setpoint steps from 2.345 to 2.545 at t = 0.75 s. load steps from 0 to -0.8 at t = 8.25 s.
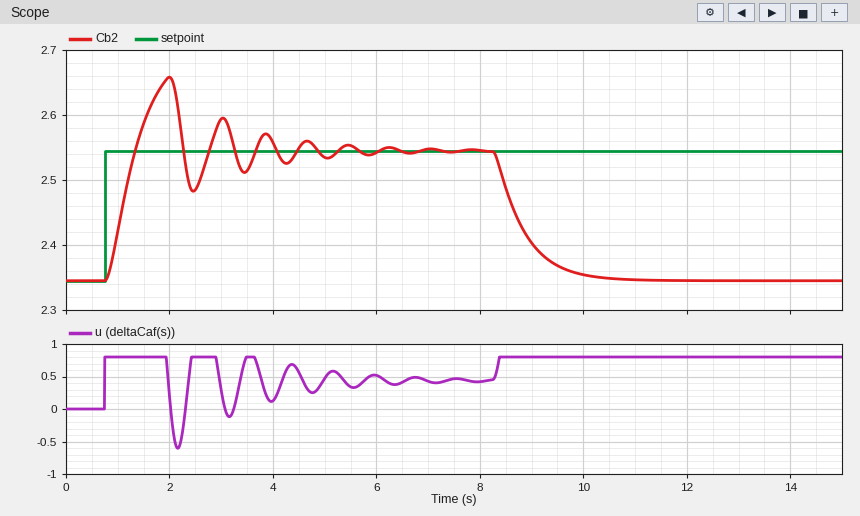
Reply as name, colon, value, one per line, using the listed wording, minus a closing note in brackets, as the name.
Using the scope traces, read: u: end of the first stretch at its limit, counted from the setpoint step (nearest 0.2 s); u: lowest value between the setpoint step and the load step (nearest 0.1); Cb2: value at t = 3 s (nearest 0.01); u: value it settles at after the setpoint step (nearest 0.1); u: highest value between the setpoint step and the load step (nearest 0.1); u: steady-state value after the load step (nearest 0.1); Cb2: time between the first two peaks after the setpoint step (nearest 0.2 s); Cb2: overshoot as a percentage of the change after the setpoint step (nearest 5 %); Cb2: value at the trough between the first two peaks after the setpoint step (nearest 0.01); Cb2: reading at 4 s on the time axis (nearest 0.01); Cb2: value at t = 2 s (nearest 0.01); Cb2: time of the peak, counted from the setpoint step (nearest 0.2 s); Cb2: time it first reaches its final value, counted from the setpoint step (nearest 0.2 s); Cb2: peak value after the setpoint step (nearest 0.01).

u: end of the first stretch at its limit, counted from the setpoint step: 1.2 s
u: lowest value between the setpoint step and the load step: -0.6
Cb2: value at t = 3 s: 2.59
u: value it settles at after the setpoint step: 0.4
u: highest value between the setpoint step and the load step: 0.8
u: steady-state value after the load step: 0.8
Cb2: time between the first two peaks after the setpoint step: 1.0 s
Cb2: overshoot as a percentage of the change after the setpoint step: 55 %
Cb2: value at the trough between the first two peaks after the setpoint step: 2.48
Cb2: reading at 4 s on the time axis: 2.56
Cb2: value at t = 2 s: 2.66
Cb2: time of the peak, counted from the setpoint step: 1.2 s
Cb2: time it first reaches its final value, counted from the setpoint step: 0.6 s
Cb2: peak value after the setpoint step: 2.66
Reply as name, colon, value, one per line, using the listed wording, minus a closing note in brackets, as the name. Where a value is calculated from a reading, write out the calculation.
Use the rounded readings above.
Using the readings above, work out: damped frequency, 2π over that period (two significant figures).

damped frequency, 2π over that period: 2π / 1 = 6.3 rad/s
